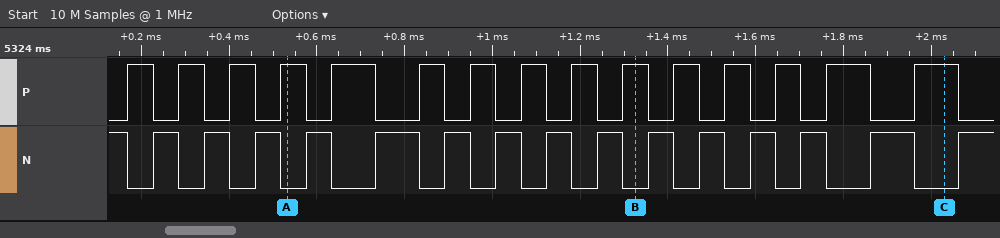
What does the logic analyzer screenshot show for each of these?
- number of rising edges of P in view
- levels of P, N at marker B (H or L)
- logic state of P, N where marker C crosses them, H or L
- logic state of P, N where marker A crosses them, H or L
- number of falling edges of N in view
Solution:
15
P=H, N=L
P=H, N=L
P=H, N=L
15
